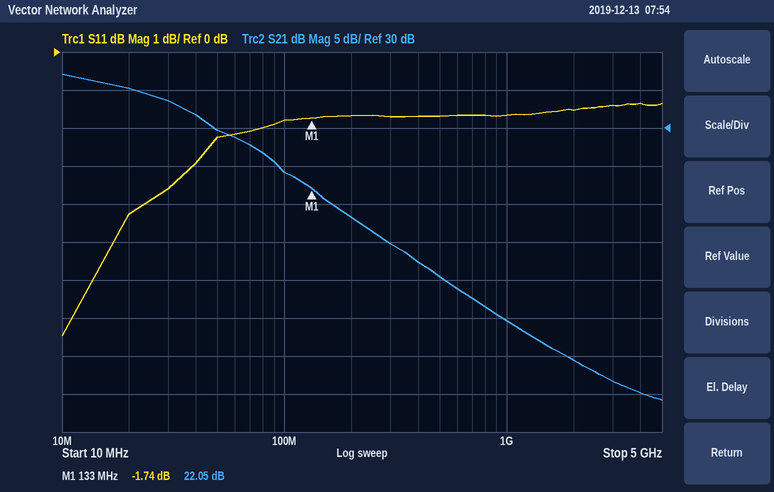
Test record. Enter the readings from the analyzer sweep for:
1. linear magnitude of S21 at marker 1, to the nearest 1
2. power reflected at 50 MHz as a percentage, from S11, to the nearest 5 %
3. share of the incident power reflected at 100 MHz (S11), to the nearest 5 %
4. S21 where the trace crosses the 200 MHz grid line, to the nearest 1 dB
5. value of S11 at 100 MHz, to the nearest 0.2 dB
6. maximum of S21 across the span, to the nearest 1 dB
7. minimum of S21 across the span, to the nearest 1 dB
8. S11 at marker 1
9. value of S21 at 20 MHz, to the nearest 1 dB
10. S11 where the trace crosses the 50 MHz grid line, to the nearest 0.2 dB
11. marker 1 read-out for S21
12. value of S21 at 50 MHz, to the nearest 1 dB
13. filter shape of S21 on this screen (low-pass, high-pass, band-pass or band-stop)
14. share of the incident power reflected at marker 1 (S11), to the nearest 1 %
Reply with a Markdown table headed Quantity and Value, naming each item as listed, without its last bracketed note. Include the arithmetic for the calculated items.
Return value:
| Quantity | Value |
|---|---|
| linear magnitude of S21 at marker 1, to the nearest 1 | 10^(22.05/20) ≈ 13 |
| power reflected at 50 MHz as a percentage, from S11, to the nearest 5 % | 10^(-2.2/10) ≈ 60 % |
| share of the incident power reflected at 100 MHz (S11), to the nearest 5 % | 10^(-1.8/10) ≈ 66.1 %, so 65 % to the nearest 5 % |
| S21 where the trace crosses the 200 MHz grid line, to the nearest 1 dB | 18 dB |
| value of S11 at 100 MHz, to the nearest 0.2 dB | -1.8 dB |
| maximum of S21 across the span, to the nearest 1 dB | 37 dB |
| minimum of S21 across the span, to the nearest 1 dB | -6 dB |
| S11 at marker 1 | -1.74 dB |
| value of S21 at 20 MHz, to the nearest 1 dB | 35 dB |
| S11 where the trace crosses the 50 MHz grid line, to the nearest 0.2 dB | -2.2 dB |
| marker 1 read-out for S21 | 22.05 dB |
| value of S21 at 50 MHz, to the nearest 1 dB | 30 dB |
| filter shape of S21 on this screen | low-pass |
| share of the incident power reflected at marker 1 (S11), to the nearest 1 % | 10^(-1.74/10) ≈ 67 % |
